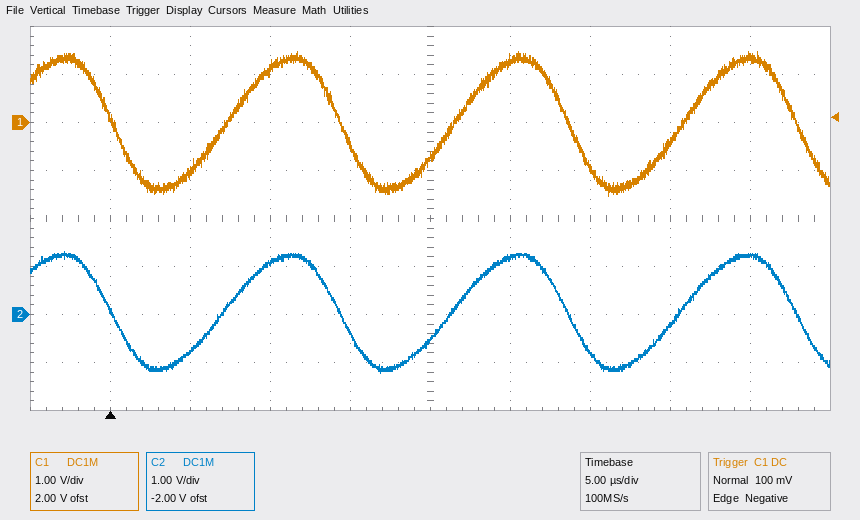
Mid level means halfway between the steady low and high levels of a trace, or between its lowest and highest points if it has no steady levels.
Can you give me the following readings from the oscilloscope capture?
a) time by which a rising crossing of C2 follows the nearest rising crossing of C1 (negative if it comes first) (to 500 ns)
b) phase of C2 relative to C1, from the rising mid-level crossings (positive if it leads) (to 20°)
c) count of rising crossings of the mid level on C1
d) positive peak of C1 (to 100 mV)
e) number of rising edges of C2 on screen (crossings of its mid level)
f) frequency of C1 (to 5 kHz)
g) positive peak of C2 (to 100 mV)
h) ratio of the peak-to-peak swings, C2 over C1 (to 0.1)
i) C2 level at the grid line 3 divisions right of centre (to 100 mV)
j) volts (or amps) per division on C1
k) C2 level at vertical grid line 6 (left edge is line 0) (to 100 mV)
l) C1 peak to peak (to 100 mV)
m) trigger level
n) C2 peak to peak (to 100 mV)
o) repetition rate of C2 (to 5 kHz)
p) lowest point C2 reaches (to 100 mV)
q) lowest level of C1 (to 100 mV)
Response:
0.0 µs
0°
3
1.5 V
3
70 kHz
1.3 V
0.8
-200 mV
1 V
1.2 V
3.0 V
100 mV
2.5 V
70 kHz
-1.2 V
-1.5 V
